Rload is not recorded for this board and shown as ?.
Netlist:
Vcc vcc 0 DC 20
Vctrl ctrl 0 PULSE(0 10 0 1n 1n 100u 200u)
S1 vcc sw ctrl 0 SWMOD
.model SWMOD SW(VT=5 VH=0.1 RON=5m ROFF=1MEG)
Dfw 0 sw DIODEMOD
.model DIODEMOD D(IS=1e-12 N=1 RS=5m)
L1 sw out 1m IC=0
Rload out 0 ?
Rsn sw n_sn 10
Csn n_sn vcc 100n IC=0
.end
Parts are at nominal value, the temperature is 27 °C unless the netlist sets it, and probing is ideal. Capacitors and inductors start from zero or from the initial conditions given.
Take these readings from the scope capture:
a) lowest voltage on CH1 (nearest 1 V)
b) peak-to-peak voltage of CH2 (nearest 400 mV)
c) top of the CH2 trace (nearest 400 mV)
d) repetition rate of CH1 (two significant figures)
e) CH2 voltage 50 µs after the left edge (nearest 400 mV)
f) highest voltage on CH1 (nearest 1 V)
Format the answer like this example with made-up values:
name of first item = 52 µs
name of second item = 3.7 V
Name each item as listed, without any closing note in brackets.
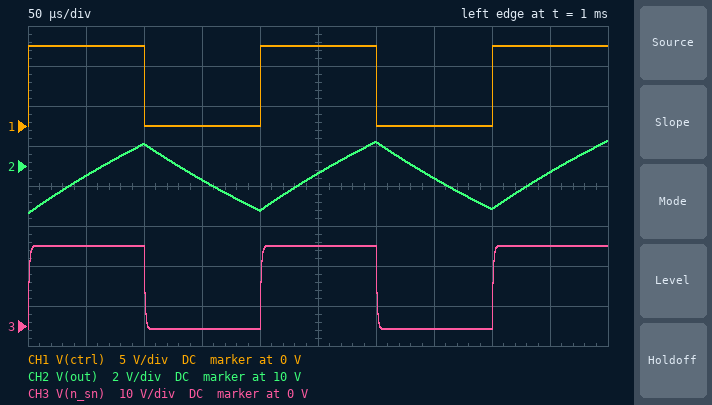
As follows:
lowest voltage on CH1 = 0 V
peak-to-peak voltage of CH2 = 3.6 V
top of the CH2 trace = 11.2 V
repetition rate of CH1 = 5.0 kHz
CH2 voltage 50 µs after the left edge = 9.6 V
highest voltage on CH1 = 10 V
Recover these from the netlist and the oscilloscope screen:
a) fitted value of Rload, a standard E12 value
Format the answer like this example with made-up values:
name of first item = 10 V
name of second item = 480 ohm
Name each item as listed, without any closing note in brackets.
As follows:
fitted value of Rload, a standard E12 value = 3.3 Ω
